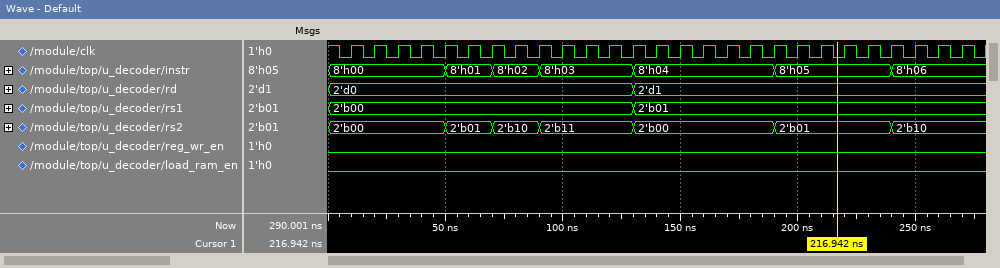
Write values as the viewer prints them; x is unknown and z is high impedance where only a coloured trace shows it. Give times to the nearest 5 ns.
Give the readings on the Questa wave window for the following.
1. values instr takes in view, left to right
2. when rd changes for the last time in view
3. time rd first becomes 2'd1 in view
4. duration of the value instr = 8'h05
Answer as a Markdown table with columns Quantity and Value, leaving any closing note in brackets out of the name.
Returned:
| Quantity | Value |
|---|---|
| values instr takes in view, left to right | 8'h00, 8'h01, 8'h02, 8'h03, 8'h04, 8'h05, 8'h06 |
| when rd changes for the last time in view | 130 ns |
| time rd first becomes 2'd1 in view | 130 ns |
| duration of the value instr = 8'h05 | 50 ns |
